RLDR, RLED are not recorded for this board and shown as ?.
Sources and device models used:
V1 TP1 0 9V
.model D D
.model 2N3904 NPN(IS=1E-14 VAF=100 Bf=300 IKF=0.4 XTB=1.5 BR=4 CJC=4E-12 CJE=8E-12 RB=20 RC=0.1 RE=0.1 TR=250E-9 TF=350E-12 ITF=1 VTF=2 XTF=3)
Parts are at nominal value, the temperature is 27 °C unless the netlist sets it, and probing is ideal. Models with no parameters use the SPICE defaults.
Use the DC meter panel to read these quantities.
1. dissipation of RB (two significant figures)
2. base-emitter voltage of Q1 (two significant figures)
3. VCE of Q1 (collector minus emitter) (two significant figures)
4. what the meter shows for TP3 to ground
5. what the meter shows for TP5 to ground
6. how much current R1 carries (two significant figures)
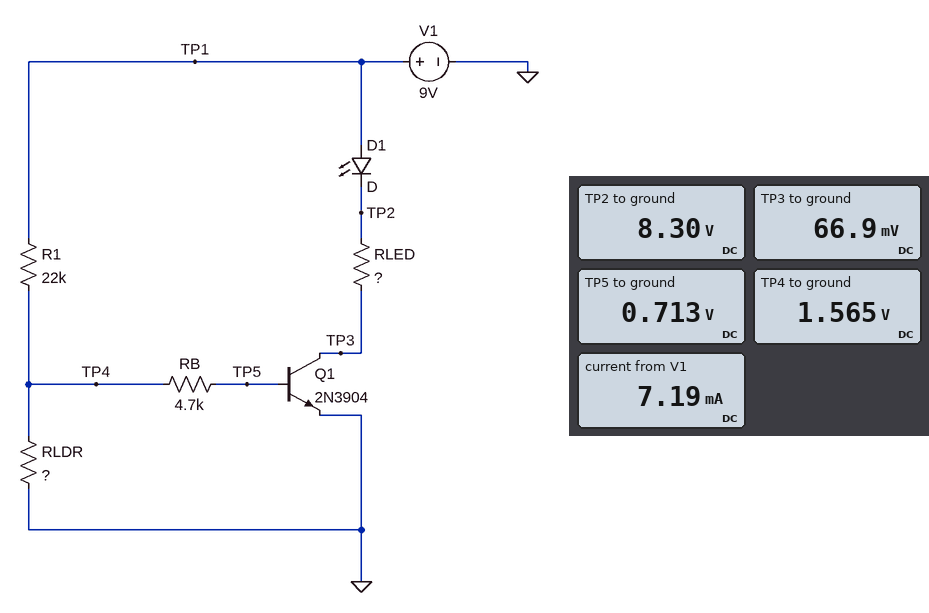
150 µW
710 mV
67 mV
66.9 mV
0.713 V
340 µA
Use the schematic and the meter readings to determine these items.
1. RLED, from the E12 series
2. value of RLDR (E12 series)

1.2 kΩ
10 kΩ
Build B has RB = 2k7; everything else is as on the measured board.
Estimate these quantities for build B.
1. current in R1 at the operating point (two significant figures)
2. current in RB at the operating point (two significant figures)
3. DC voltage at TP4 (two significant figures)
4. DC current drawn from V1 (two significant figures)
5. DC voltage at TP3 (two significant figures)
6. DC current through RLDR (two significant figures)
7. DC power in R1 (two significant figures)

350 µA
220 µA
1.3 V
7.2 mA
62 mV
130 µA
2.7 mW
